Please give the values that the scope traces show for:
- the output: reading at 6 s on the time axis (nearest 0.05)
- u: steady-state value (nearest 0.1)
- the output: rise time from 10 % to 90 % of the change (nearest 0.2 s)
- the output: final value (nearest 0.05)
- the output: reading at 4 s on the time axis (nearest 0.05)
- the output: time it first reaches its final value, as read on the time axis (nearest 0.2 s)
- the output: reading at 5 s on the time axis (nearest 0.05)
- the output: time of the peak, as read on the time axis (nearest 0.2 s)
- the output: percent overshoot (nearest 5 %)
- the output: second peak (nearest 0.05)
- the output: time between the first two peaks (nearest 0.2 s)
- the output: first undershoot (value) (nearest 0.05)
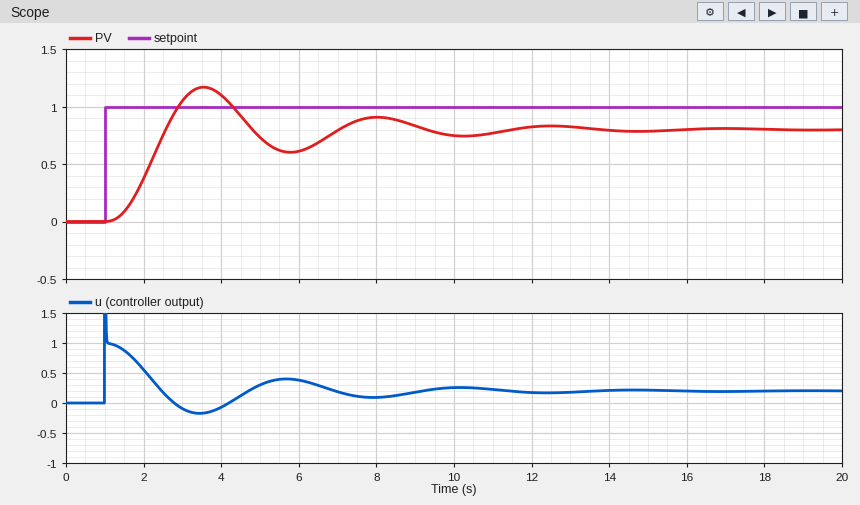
0.60
0.2
1.0 s
0.80
1.10
2.6 s
0.75
3.6 s
45 %
0.90
4.4 s
0.60
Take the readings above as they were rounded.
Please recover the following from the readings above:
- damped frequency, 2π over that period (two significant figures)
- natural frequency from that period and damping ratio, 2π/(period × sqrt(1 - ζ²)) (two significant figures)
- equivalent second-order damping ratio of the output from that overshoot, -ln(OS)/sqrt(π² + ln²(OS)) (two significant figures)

1.4 rad/s
1.5 rad/s
0.25
